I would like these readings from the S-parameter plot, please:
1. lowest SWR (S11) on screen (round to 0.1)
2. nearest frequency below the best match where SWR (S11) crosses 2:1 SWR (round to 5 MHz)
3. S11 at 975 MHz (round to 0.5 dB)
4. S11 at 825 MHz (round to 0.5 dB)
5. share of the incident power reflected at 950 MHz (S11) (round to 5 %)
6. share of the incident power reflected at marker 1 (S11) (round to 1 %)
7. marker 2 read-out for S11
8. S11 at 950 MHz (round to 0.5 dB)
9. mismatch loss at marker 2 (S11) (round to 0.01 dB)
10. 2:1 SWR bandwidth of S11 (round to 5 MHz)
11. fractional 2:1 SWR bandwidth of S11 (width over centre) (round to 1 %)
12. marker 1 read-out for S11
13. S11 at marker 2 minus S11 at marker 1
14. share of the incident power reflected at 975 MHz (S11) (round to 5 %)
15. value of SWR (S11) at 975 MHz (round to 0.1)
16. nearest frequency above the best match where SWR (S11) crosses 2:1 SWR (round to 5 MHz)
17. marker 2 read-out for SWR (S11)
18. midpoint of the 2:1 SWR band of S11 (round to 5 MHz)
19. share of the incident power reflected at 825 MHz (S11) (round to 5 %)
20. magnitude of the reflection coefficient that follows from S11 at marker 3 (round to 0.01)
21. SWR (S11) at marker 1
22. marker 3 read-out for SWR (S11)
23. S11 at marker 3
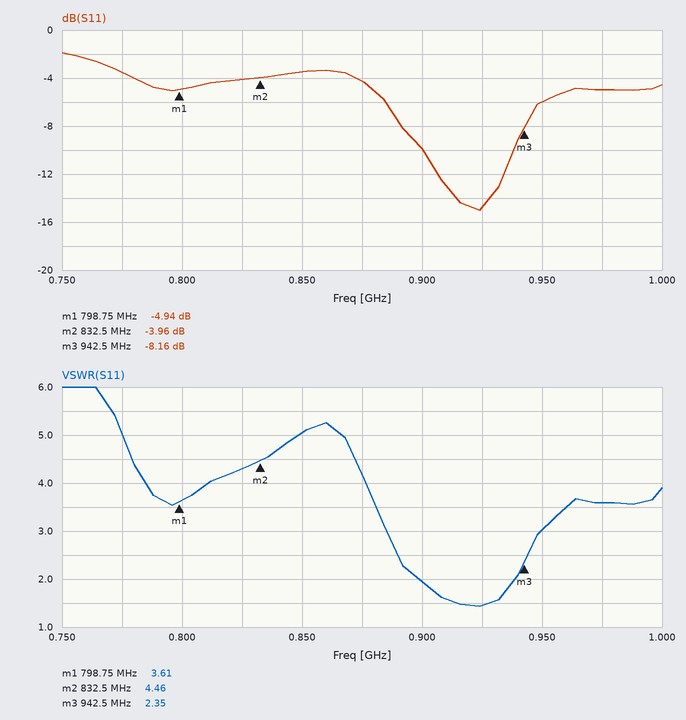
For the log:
1.4
900 MHz
-5.0 dB
-4.0 dB
25 %
32 %
-3.96 dB
-6.0 dB
2.23 dB
40 MHz
4 %
-4.94 dB
0.98 dB
30 %
3.6
940 MHz
4.46
920 MHz
40 %
0.39
3.61
2.35
-8.16 dB
